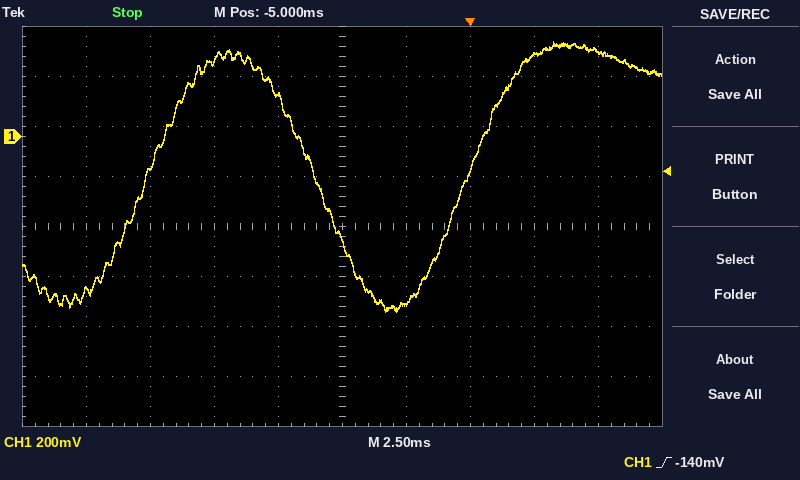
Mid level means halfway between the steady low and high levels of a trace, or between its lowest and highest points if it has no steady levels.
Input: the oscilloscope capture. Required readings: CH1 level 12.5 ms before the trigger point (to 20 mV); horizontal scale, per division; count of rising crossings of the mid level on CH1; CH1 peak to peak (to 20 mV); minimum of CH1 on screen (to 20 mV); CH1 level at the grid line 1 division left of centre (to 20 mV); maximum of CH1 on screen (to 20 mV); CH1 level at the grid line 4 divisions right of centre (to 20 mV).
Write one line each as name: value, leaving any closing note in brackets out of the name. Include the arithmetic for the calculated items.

CH1 level 12.5 ms before the trigger point: -120 mV
horizontal scale, per division: 2.5 ms
count of rising crossings of the mid level on CH1: 2
CH1 peak to peak: 380 mV − (-700 mV) = 1.08 V
minimum of CH1 on screen: -700 mV
CH1 level at the grid line 1 division left of centre: 160 mV
maximum of CH1 on screen: 380 mV
CH1 level at the grid line 4 divisions right of centre: 340 mV
